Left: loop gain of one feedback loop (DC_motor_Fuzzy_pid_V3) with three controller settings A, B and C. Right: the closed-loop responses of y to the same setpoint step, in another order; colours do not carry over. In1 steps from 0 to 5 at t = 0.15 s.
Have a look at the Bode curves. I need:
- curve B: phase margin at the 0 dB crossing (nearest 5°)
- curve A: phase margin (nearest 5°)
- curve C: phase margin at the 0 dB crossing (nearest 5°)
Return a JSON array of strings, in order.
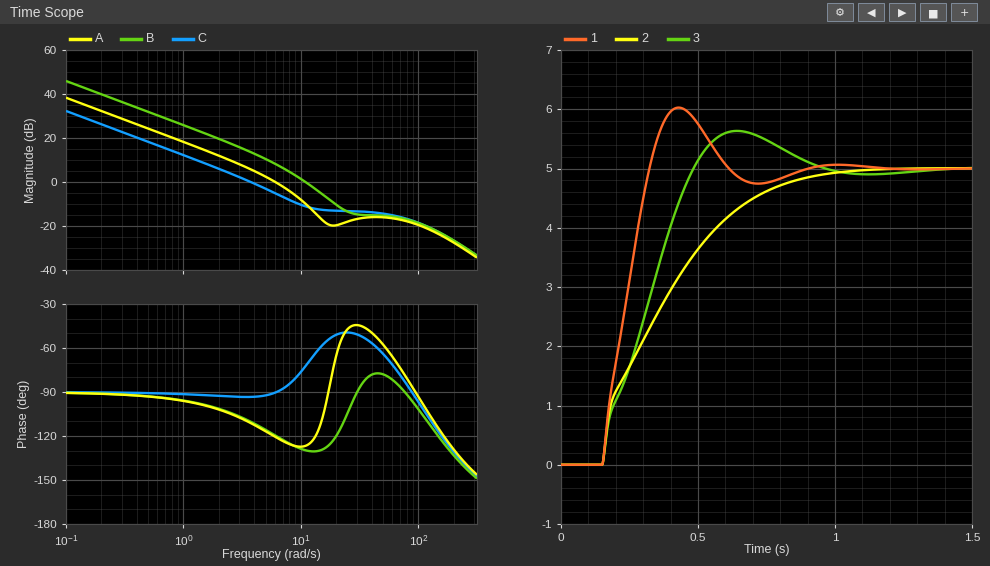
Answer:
["50°", "60°", "85°"]
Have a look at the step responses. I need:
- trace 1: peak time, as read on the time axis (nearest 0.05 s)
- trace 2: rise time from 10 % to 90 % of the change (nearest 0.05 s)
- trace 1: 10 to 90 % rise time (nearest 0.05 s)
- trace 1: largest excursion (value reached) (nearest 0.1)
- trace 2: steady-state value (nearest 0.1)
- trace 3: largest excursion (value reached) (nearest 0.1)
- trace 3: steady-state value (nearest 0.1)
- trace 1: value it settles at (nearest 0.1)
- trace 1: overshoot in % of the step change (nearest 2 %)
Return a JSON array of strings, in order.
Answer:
["0.45 s", "0.55 s", "0.15 s", "6.0", "5.0", "5.6", "5.0", "5.0", "20 %"]
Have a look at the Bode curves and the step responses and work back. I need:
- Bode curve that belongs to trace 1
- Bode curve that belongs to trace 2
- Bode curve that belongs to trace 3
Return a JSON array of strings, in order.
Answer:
["B", "C", "A"]
